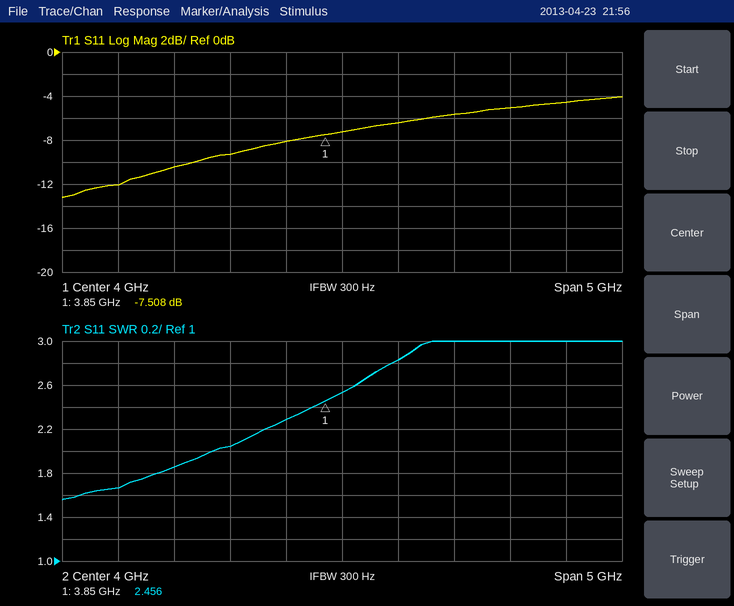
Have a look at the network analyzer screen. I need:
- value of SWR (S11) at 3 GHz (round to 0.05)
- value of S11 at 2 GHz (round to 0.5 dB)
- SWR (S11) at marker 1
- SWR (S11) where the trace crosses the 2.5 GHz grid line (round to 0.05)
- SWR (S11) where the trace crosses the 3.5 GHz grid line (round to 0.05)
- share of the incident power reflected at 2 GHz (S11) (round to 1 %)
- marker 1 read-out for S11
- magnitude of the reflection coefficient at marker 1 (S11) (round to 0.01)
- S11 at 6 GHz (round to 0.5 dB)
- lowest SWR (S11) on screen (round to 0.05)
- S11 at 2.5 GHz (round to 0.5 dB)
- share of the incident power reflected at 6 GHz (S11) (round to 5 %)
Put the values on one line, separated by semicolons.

2.05; -12.0 dB; 2.456; 1.85; 2.30; 6 %; -7.508 dB; 0.42; -4.5 dB; 1.55; -10.5 dB; 35 %
